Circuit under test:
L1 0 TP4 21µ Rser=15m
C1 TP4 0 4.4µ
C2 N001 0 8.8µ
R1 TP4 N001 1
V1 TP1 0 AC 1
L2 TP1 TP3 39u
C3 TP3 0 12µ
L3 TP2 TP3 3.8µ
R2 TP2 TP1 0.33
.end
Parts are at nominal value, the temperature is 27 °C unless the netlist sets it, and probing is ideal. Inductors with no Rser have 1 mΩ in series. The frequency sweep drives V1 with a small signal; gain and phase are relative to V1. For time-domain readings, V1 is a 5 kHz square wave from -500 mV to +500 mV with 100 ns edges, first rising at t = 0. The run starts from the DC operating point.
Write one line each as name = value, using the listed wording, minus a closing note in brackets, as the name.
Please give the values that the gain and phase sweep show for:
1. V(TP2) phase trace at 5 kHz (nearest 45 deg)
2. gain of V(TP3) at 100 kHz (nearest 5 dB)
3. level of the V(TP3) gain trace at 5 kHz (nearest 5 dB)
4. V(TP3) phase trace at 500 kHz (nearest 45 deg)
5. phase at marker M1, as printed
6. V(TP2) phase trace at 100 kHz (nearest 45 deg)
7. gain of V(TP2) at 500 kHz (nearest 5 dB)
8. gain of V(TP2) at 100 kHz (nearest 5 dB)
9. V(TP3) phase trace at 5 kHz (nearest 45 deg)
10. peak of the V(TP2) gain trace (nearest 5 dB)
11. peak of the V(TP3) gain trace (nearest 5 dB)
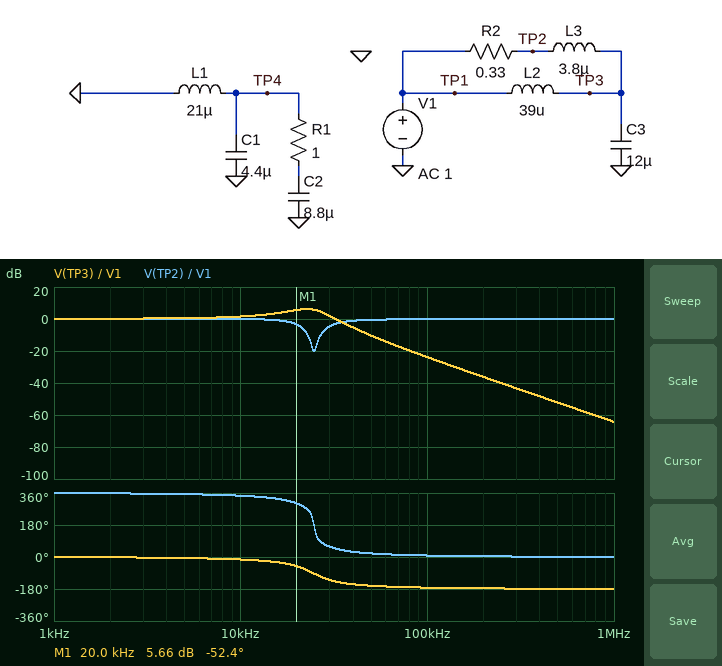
V(TP2) phase trace at 5 kHz = 360 deg
gain of V(TP3) at 100 kHz = -25 dB
level of the V(TP3) gain trace at 5 kHz = 0 dB
V(TP3) phase trace at 500 kHz = -180 deg
phase at marker M1, as printed = -52.4 deg
V(TP2) phase trace at 100 kHz = 0 deg
gain of V(TP2) at 500 kHz = 0 dB
gain of V(TP2) at 100 kHz = 0 dB
V(TP3) phase trace at 5 kHz = 0 deg
peak of the V(TP2) gain trace = 0 dB
peak of the V(TP3) gain trace = 5 dB
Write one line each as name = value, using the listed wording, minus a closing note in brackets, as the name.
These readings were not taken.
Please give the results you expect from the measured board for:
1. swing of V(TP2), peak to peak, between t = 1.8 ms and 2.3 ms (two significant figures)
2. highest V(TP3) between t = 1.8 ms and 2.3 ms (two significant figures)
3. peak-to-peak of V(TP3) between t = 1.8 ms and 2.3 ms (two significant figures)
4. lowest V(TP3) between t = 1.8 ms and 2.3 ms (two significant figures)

swing of V(TP2), peak to peak, between t = 1.8 ms and 2.3 ms = 1.4 V
highest V(TP3) between t = 1.8 ms and 2.3 ms = 960 mV
peak-to-peak of V(TP3) between t = 1.8 ms and 2.3 ms = 1.9 V
lowest V(TP3) between t = 1.8 ms and 2.3 ms = -960 mV
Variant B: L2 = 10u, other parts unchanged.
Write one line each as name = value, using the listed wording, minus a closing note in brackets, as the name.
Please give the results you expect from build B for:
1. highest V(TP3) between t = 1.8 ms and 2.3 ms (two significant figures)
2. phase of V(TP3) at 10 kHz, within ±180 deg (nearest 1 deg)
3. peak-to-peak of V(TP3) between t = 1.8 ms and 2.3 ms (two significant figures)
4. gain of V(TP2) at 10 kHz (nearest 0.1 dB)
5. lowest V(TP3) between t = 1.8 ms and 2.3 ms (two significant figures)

highest V(TP3) between t = 1.8 ms and 2.3 ms = 1.1 V
phase of V(TP3) at 10 kHz, within ±180 deg = -8 deg
peak-to-peak of V(TP3) between t = 1.8 ms and 2.3 ms = 2.3 V
gain of V(TP2) at 10 kHz = 0.5 dB
lowest V(TP3) between t = 1.8 ms and 2.3 ms = -1.1 V
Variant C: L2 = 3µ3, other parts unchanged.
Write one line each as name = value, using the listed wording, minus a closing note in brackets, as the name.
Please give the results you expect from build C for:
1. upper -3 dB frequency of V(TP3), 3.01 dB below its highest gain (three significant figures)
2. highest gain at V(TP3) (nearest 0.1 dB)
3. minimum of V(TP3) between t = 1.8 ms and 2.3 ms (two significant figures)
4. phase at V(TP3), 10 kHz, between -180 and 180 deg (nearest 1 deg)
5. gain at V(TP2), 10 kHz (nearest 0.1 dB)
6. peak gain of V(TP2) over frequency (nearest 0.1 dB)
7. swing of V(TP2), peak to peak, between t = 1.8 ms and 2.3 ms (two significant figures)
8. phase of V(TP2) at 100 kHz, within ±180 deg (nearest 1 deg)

upper -3 dB frequency of V(TP3), 3.01 dB below its highest gain = 36.6 kHz
highest gain at V(TP3) = 15.2 dB
minimum of V(TP3) between t = 1.8 ms and 2.3 ms = -1.4 V
phase at V(TP3), 10 kHz, between -180 and 180 deg = -2 deg
gain at V(TP2), 10 kHz = 0.5 dB
peak gain of V(TP2) over frequency = 2.6 dB
swing of V(TP2), peak to peak, between t = 1.8 ms and 2.3 ms = 1.7 V
phase of V(TP2) at 100 kHz, within ±180 deg = 9 deg
